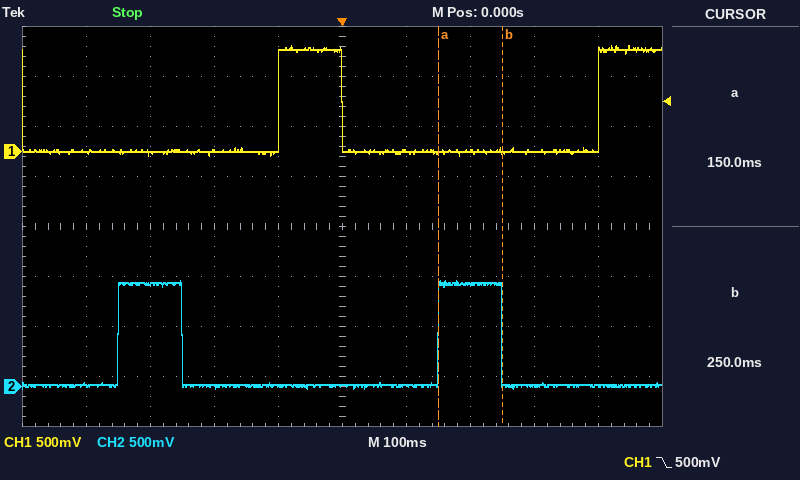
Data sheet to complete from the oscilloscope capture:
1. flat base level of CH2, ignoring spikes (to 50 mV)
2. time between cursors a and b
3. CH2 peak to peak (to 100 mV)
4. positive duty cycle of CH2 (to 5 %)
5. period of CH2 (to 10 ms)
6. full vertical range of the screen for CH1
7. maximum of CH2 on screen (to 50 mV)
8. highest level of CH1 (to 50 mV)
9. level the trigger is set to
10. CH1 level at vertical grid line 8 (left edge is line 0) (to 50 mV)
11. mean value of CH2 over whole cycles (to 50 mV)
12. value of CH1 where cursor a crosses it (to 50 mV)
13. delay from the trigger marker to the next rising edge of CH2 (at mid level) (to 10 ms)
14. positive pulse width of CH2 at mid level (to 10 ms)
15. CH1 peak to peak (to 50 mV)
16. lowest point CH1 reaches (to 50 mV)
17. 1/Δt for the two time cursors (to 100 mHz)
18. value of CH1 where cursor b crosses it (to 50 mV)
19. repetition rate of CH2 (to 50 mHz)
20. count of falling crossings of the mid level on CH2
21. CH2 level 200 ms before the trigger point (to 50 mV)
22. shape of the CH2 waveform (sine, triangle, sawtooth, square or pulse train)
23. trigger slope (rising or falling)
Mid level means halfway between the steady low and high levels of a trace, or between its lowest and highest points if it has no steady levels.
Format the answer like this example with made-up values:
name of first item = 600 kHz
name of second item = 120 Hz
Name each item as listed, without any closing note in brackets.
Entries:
flat base level of CH2, ignoring spikes = 0 mV
time between cursors a and b = 100 ms
CH2 peak to peak = 1.10 V
positive duty cycle of CH2 = 20 %
period of CH2 = 500 ms
full vertical range of the screen for CH1 = 4 V
maximum of CH2 on screen = 1.05 V
highest level of CH1 = 1.05 V
level the trigger is set to = 500 mV
CH1 level at vertical grid line 8 (left edge is line 0) = 0 mV
mean value of CH2 over whole cycles = 200 mV
value of CH1 where cursor a crosses it = 0 mV
delay from the trigger marker to the next rising edge of CH2 (at mid level) = 150 ms
positive pulse width of CH2 at mid level = 100 ms
CH1 peak to peak = 1.10 V
lowest point CH1 reaches = -50 mV
1/Δt for the two time cursors = 10.0 Hz
value of CH1 where cursor b crosses it = 0 mV
repetition rate of CH2 = 2.00 Hz
count of falling crossings of the mid level on CH2 = 2
CH2 level 200 ms before the trigger point = 0 mV
shape of the CH2 waveform = pulse train
trigger slope = falling
